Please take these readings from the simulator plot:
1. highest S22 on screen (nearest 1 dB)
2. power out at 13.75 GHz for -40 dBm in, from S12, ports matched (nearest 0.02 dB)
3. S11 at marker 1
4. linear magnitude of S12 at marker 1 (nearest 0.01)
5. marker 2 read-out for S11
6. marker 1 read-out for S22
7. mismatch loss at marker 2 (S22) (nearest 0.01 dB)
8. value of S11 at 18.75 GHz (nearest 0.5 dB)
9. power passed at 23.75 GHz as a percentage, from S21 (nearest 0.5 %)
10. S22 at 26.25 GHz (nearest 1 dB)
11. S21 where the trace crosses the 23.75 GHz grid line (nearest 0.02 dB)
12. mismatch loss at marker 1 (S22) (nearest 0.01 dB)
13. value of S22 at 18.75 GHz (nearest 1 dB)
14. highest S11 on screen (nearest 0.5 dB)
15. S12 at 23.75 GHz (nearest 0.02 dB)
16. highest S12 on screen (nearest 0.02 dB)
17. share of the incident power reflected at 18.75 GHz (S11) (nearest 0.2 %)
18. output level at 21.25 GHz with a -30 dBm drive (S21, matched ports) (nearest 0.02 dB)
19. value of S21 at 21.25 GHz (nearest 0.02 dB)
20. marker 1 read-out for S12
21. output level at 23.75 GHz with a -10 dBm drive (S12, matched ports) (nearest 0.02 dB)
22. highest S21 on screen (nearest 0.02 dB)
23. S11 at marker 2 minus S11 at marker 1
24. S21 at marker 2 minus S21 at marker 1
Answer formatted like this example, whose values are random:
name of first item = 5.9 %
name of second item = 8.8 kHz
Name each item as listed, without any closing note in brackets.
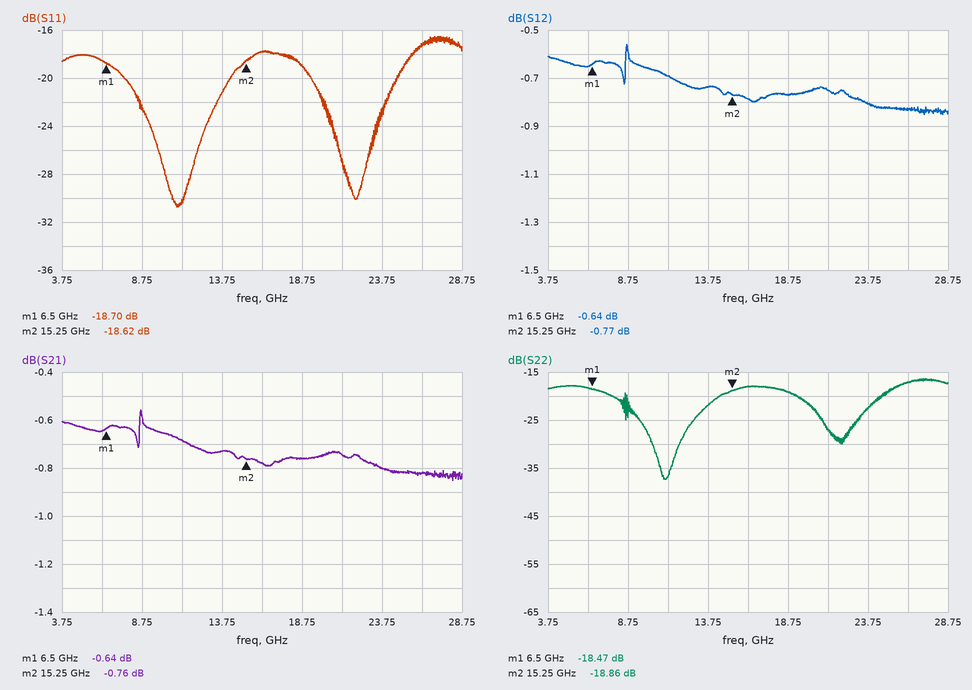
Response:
highest S22 on screen = -16 dB
power out at 13.75 GHz for -40 dBm in, from S12, ports matched = -40.74 dBm
S11 at marker 1 = -18.70 dB
linear magnitude of S12 at marker 1 = 0.93
marker 2 read-out for S11 = -18.62 dB
marker 1 read-out for S22 = -18.47 dB
mismatch loss at marker 2 (S22) = 0.06 dB
value of S11 at 18.75 GHz = -19.0 dB
power passed at 23.75 GHz as a percentage, from S21 = 83.0 %
S22 at 26.25 GHz = -17 dB
S21 where the trace crosses the 23.75 GHz grid line = -0.80 dB
mismatch loss at marker 1 (S22) = 0.06 dB
value of S22 at 18.75 GHz = -19 dB
highest S11 on screen = -16.5 dB
S12 at 23.75 GHz = -0.80 dB
highest S12 on screen = -0.56 dB
share of the incident power reflected at 18.75 GHz (S11) = 1.2 %
output level at 21.25 GHz with a -30 dBm drive (S21, matched ports) = -30.74 dBm
value of S21 at 21.25 GHz = -0.74 dB
marker 1 read-out for S12 = -0.64 dB
output level at 23.75 GHz with a -10 dBm drive (S12, matched ports) = -10.80 dBm
highest S21 on screen = -0.56 dB
S11 at marker 2 minus S11 at marker 1 = 0.08 dB
S21 at marker 2 minus S21 at marker 1 = -0.12 dB
